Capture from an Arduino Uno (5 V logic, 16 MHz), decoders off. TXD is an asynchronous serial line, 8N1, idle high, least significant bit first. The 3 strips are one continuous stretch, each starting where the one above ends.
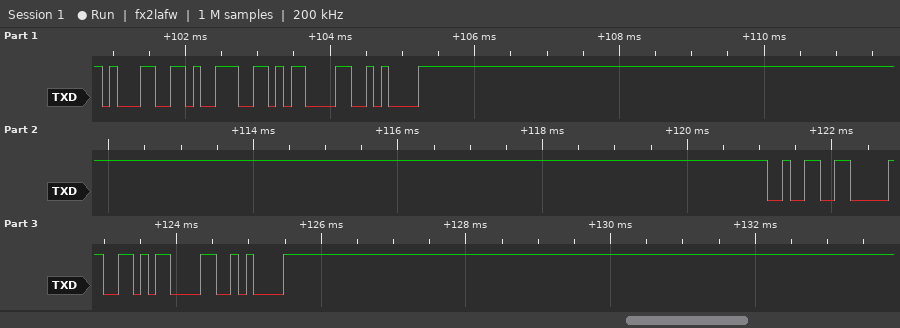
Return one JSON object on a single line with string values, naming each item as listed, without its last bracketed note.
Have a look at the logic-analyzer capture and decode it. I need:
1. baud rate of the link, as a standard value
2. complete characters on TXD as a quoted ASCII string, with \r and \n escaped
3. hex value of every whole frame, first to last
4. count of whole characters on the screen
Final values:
{"baud rate of the link, as a standard value": "9600 baud", "complete characters on TXD as a quoted ASCII string, with \\r and \\n escaped": "\"19\\r\\n20\\r\\n\"", "hex value of every whole frame, first to last": "0x31 0x39 0x0D 0x0A 0x32 0x30 0x0D 0x0A", "count of whole characters on the screen": "8"}
